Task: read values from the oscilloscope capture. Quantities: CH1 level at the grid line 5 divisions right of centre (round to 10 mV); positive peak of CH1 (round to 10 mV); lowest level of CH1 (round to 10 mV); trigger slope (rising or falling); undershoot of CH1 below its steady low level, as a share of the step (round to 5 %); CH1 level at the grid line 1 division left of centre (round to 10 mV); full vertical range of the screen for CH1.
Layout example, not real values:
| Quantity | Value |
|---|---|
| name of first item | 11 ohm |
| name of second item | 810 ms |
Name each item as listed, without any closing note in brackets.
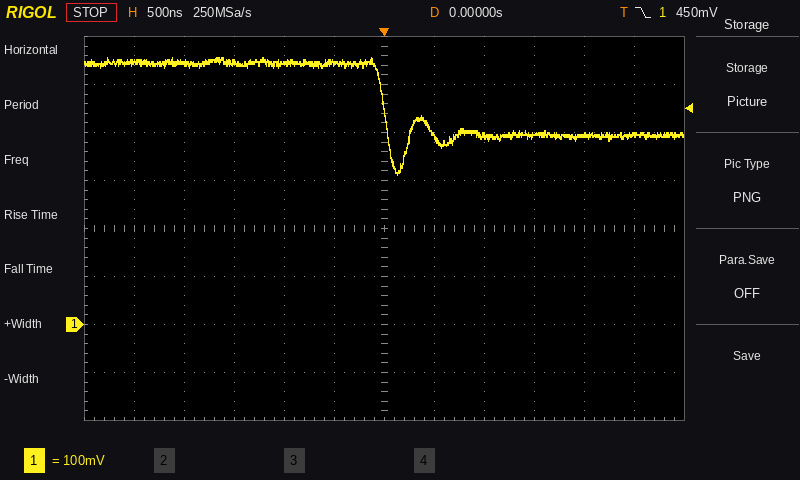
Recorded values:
| Quantity | Value |
|---|---|
| CH1 level at the grid line 5 divisions right of centre | 400 mV |
| positive peak of CH1 | 560 mV |
| lowest level of CH1 | 310 mV |
| trigger slope | falling |
| undershoot of CH1 below its steady low level, as a share of the step | 55 % |
| CH1 level at the grid line 1 division left of centre | 550 mV |
| full vertical range of the screen for CH1 | 800 mV |
